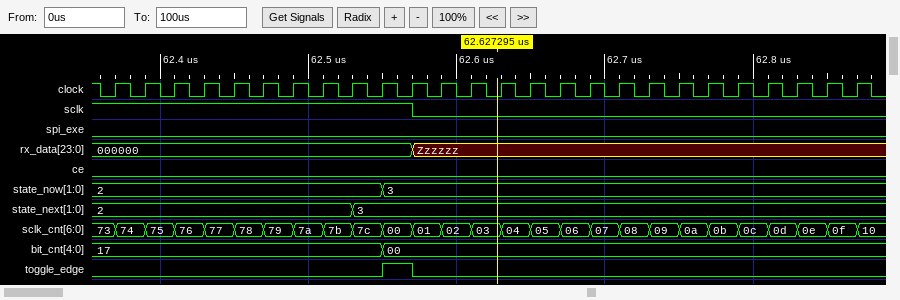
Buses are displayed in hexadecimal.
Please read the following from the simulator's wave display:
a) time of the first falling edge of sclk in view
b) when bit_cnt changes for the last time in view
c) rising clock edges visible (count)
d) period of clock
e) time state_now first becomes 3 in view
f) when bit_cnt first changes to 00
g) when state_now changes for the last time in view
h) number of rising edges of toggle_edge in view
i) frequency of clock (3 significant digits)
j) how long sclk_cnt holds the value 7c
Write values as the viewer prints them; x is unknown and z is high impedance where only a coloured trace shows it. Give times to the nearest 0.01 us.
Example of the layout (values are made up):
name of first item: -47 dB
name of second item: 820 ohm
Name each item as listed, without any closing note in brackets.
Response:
time of the first falling edge of sclk in view: 62.57 us
when bit_cnt changes for the last time in view: 62.55 us
rising clock edges visible: 26
period of clock: 0.02 us
time state_now first becomes 3 in view: 62.55 us
when bit_cnt first changes to 00: 62.55 us
when state_now changes for the last time in view: 62.55 us
number of rising edges of toggle_edge in view: 1
frequency of clock: 50.0 MHz
how long sclk_cnt holds the value 7c: 0.02 us
